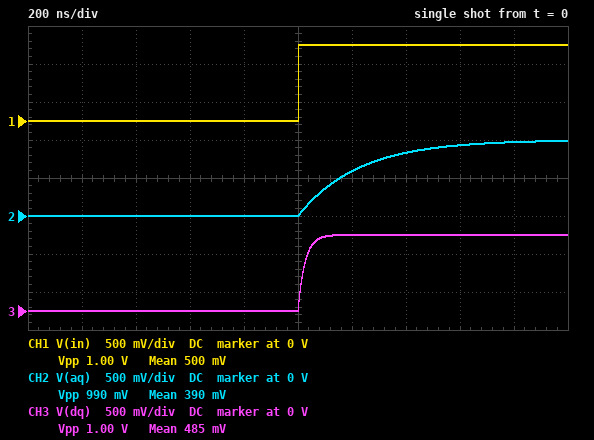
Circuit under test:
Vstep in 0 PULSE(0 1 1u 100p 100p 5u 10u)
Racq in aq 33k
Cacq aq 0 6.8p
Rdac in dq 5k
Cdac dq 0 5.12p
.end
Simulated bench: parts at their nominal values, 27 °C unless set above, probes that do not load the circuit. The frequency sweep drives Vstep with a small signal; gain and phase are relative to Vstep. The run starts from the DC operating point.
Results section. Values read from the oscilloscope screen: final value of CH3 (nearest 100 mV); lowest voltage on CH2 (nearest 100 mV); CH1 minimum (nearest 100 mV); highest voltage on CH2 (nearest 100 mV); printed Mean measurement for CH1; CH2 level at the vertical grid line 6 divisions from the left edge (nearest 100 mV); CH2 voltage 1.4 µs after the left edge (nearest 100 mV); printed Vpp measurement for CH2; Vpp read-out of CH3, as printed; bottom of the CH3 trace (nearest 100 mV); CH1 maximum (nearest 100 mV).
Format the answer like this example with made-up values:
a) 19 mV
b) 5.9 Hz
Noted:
a) 1.0 V
b) 0 V
c) 0 V
d) 1.0 V
e) 500 mV
f) 600 mV
g) 800 mV
h) 990 mV
i) 1.00 V
j) 0 V
k) 1.0 V
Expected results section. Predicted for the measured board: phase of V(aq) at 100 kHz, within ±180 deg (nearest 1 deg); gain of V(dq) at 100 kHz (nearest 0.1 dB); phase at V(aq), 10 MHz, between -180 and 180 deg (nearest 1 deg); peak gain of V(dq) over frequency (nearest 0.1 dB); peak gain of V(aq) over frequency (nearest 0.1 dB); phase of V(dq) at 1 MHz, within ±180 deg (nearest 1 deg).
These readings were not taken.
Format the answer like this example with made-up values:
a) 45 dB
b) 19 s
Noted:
a) -8 deg
b) 0 dB
c) -86 deg
d) 0 dB
e) 0 dB
f) -9 deg
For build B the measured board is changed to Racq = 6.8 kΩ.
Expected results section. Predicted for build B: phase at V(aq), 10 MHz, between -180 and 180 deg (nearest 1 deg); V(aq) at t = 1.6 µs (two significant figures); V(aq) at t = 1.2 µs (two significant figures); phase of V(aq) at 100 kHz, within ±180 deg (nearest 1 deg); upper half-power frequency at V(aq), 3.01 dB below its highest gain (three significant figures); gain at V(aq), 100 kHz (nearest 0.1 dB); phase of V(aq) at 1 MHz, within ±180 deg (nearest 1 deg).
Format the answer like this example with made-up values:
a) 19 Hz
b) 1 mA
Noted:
a) -71 deg
b) 1.0 V
c) 990 mV
d) -2 deg
e) 3.44 MHz
f) 0 dB
g) -16 deg
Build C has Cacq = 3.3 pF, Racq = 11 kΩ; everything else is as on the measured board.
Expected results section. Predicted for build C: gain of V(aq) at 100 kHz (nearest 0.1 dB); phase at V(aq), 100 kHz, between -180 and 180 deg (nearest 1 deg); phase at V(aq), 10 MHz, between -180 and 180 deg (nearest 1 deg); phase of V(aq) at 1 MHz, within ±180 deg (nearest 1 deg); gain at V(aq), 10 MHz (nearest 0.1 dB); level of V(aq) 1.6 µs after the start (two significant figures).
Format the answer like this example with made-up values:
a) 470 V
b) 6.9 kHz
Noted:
a) 0 dB
b) -1 deg
c) -66 deg
d) -13 deg
e) -7.9 dB
f) 1.0 V
